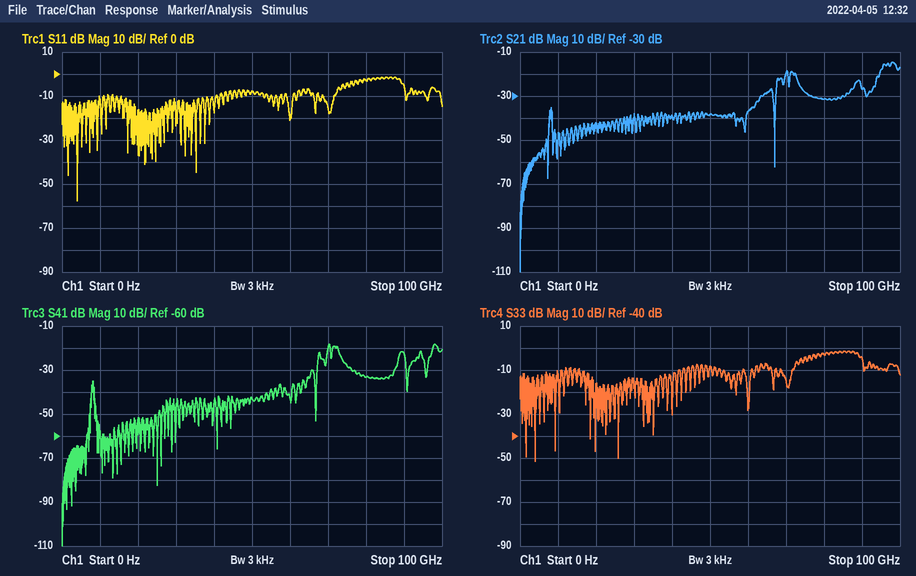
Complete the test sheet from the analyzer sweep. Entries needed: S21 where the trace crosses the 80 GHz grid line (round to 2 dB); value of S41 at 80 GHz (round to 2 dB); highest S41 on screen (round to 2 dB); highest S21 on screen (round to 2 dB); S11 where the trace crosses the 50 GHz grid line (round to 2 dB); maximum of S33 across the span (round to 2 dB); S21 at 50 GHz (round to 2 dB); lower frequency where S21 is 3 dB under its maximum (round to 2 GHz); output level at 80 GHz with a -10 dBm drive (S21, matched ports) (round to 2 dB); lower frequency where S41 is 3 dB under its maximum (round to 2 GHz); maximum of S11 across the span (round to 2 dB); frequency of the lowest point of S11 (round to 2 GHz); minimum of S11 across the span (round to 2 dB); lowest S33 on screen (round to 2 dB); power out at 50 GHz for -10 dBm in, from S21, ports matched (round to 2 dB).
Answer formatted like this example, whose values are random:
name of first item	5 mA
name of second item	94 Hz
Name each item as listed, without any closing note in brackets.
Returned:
S21 where the trace crosses the 80 GHz grid line	-32 dB
value of S41 at 80 GHz	-34 dB
highest S41 on screen	-18 dB
highest S21 on screen	-14 dB
S11 where the trace crosses the 50 GHz grid line	-8 dB
maximum of S33 across the span	-2 dB
S21 at 50 GHz	-38 dB
lower frequency where S21 is 3 dB under its maximum	96 GHz
output level at 80 GHz with a -10 dBm drive (S21, matched ports)	-42 dBm
lower frequency where S41 is 3 dB under its maximum	70 GHz
maximum of S11 across the span	-2 dB
frequency of the lowest point of S11	4 GHz
minimum of S11 across the span	-58 dB
lowest S33 on screen	-52 dB
power out at 50 GHz for -10 dBm in, from S21, ports matched	-48 dBm
